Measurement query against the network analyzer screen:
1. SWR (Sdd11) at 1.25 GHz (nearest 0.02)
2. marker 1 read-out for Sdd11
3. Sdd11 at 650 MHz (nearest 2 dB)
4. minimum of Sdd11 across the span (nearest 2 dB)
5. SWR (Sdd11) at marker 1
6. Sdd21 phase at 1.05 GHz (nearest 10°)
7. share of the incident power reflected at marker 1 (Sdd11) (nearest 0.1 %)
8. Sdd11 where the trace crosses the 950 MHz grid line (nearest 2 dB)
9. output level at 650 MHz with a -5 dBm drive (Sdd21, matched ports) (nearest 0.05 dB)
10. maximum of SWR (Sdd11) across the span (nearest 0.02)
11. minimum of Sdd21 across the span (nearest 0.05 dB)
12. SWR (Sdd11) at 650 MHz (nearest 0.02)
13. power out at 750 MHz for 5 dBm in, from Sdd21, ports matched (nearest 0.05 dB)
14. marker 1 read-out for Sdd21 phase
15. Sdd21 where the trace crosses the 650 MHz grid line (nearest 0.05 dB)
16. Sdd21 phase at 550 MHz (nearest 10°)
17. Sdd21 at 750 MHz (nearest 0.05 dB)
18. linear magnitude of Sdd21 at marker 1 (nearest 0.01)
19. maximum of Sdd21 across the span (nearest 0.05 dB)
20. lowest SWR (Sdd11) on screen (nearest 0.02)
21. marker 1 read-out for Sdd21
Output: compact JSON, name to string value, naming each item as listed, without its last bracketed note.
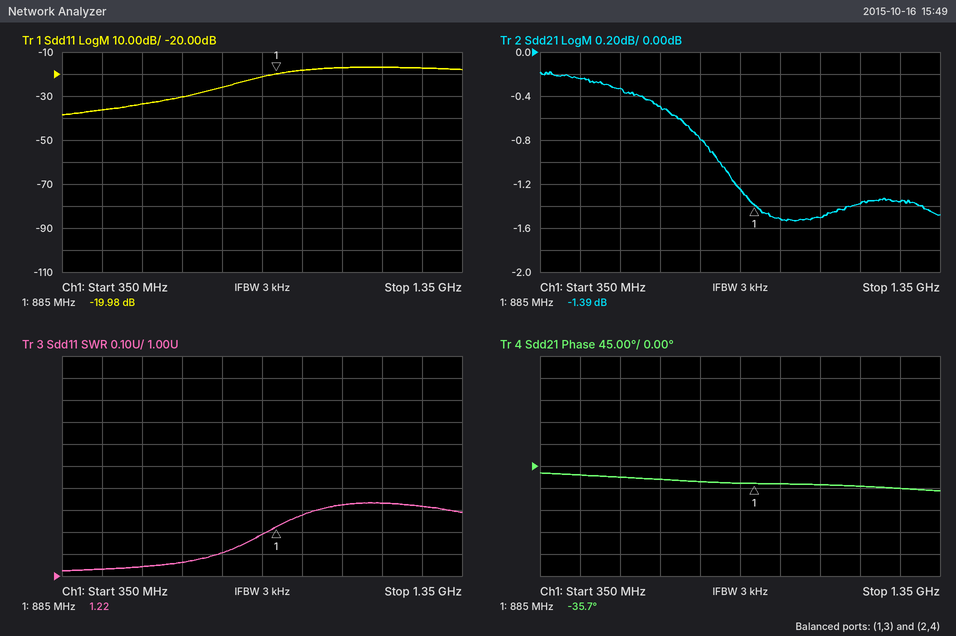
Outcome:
{"SWR (Sdd11) at 1.25 GHz": "1.32", "marker 1 read-out for Sdd11": "-19.98 dB", "Sdd11 at 650 MHz": "-30 dB", "minimum of Sdd11 across the span": "-38 dB", "SWR (Sdd11) at marker 1": "1.22", "Sdd21 phase at 1.05 GHz": "-40°", "share of the incident power reflected at marker 1 (Sdd11)": "1.0 %", "Sdd11 where the trace crosses the 950 MHz grid line": "-18 dB", "output level at 650 MHz with a -5 dBm drive (Sdd21, matched ports)": "-5.50 dBm", "maximum of SWR (Sdd11) across the span": "1.34", "minimum of Sdd21 across the span": "-1.55 dB", "SWR (Sdd11) at 650 MHz": "1.06", "power out at 750 MHz for 5 dBm in, from Sdd21, ports matched": "4.20 dBm", "marker 1 read-out for Sdd21 phase": "-35.7°", "Sdd21 where the trace crosses the 650 MHz grid line": "-0.50 dB", "Sdd21 phase at 550 MHz": "-20°", "Sdd21 at 750 MHz": "-0.80 dB", "linear magnitude of Sdd21 at marker 1": "0.85", "maximum of Sdd21 across the span": "-0.20 dB", "lowest SWR (Sdd11) on screen": "1.02", "marker 1 read-out for Sdd21": "-1.39 dB"}
